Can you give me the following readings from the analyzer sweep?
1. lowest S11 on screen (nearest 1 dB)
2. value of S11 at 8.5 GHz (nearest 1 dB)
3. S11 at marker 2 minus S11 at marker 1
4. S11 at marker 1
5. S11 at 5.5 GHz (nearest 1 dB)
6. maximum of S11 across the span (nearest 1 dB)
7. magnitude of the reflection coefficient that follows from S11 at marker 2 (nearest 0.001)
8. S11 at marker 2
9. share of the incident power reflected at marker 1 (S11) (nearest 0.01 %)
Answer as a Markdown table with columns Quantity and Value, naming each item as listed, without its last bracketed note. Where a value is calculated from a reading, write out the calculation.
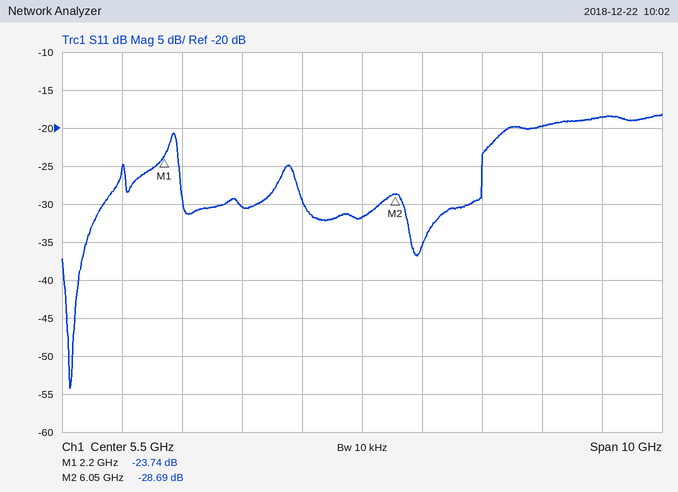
| Quantity | Value |
|---|---|
| lowest S11 on screen | -54 dB |
| value of S11 at 8.5 GHz | -20 dB |
| S11 at marker 2 minus S11 at marker 1 | -28.69 − (-23.74) = -4.95 dB |
| S11 at marker 1 | -23.74 dB |
| S11 at 5.5 GHz | -32 dB |
| maximum of S11 across the span | -18 dB |
| magnitude of the reflection coefficient that follows from S11 at marker 2 | 10^(-28.69/20) ≈ 0.037 |
| S11 at marker 2 | -28.69 dB |
| share of the incident power reflected at marker 1 (S11) | 10^(-23.74/10) ≈ 0.42 % |
